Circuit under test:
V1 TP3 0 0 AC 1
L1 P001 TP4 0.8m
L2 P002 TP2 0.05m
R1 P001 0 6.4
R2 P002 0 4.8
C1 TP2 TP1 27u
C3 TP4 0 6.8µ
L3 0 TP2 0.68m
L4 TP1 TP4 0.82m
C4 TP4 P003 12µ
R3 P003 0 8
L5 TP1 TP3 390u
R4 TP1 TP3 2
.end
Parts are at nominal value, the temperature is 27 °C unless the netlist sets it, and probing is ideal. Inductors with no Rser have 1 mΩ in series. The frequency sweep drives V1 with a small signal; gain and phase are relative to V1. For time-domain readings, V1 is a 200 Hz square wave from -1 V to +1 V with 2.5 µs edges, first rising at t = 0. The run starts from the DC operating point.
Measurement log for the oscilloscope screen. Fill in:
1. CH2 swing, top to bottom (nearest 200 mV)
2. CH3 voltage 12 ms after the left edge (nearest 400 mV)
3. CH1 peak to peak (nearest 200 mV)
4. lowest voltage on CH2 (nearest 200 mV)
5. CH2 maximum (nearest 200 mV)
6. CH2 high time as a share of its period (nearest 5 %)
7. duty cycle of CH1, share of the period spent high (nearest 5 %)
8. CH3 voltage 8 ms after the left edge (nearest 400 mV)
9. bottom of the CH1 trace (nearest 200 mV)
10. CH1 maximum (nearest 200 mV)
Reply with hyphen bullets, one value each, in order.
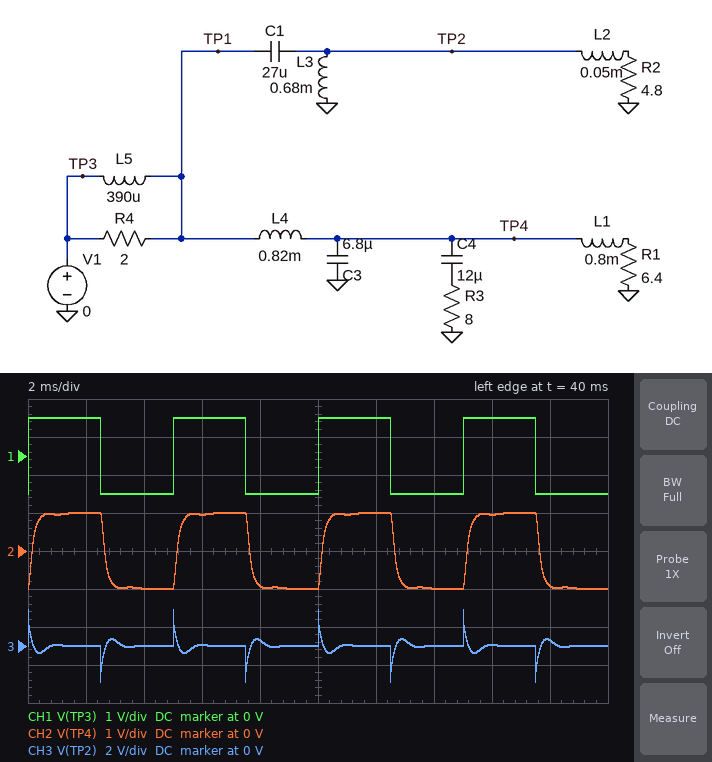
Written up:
- 2.0 V
- 0 V
- 2.0 V
- -1.0 V
- 1.0 V
- 50 %
- 50 %
- 400 mV
- -1.0 V
- 1.0 V
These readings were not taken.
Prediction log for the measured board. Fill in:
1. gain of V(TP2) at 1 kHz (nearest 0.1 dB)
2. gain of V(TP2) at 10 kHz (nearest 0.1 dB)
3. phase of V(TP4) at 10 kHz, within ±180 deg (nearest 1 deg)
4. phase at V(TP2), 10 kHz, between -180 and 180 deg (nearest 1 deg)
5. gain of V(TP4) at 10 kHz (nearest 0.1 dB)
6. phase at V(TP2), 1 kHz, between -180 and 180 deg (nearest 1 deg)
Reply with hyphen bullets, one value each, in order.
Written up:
- -3.8 dB
- -2.2 dB
- -153 deg
- 15 deg
- -29.6 dB
- 90 deg
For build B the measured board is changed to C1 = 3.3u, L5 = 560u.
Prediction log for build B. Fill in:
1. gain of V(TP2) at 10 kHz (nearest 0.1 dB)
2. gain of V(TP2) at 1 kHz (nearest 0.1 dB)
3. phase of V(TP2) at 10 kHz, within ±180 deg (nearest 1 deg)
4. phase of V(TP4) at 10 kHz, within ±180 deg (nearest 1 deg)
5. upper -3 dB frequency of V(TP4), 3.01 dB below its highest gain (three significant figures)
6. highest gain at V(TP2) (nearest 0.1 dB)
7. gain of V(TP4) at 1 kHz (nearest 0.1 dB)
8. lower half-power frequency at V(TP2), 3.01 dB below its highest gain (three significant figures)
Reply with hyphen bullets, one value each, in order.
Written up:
- -1.4 dB
- -24.9 dB
- 53 deg
- -169 deg
- 1.86 kHz
- 0.2 dB
- -2.4 dB
- 7.79 kHz
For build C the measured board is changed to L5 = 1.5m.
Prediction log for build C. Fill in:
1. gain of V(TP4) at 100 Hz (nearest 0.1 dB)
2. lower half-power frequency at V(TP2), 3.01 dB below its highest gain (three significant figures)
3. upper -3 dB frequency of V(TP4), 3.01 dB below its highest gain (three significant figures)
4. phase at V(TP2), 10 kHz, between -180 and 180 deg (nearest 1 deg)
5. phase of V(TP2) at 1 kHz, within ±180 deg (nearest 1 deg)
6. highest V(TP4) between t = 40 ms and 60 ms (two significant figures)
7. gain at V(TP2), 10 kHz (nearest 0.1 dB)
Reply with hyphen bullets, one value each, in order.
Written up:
- -0.5 dB
- 2.57 kHz
- 798 Hz
- 16 deg
- 94 deg
- 960 mV
- -2.1 dB
